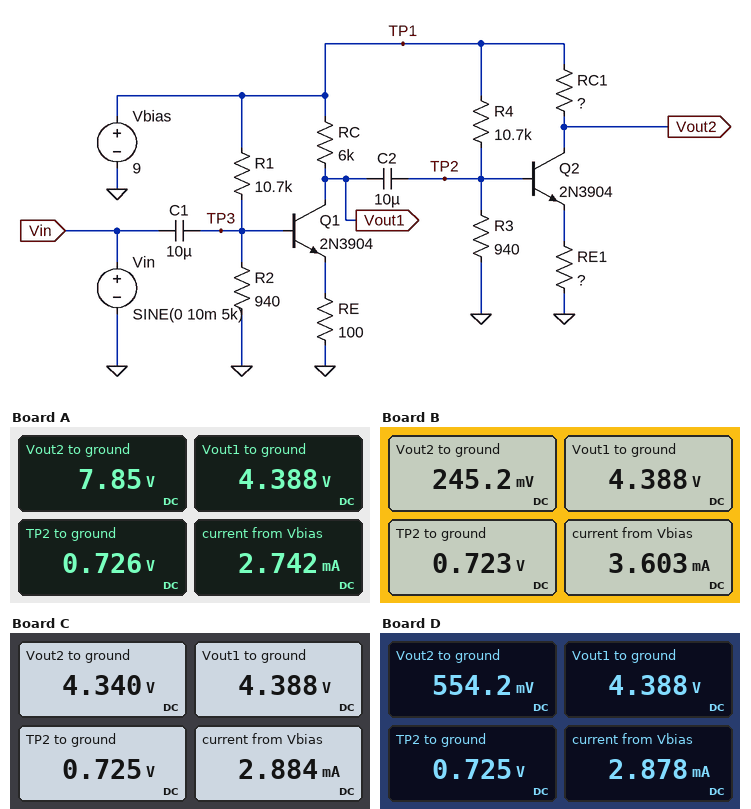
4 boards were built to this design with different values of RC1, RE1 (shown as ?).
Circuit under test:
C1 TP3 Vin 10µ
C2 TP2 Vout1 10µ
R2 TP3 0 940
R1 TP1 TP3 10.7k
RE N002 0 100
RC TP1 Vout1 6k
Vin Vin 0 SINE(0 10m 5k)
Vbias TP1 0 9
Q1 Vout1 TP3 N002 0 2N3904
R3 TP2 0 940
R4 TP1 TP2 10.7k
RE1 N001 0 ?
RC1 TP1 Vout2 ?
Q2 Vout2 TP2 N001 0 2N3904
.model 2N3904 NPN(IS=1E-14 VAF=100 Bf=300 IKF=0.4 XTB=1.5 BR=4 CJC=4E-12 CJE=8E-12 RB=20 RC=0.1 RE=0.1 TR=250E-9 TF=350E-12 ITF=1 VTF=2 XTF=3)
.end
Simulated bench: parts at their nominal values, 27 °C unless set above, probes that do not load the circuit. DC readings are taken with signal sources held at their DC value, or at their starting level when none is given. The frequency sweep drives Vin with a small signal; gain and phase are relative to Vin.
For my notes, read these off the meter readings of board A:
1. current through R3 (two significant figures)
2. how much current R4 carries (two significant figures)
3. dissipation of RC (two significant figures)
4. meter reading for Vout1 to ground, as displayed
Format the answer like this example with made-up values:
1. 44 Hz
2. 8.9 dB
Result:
1. 770 µA
2. 770 µA
3. 3.5 mW
4. 4.388 V
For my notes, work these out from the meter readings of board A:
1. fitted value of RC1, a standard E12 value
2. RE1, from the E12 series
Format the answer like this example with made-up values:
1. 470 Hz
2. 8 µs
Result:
1. 2.7 kΩ
2. 220 Ω
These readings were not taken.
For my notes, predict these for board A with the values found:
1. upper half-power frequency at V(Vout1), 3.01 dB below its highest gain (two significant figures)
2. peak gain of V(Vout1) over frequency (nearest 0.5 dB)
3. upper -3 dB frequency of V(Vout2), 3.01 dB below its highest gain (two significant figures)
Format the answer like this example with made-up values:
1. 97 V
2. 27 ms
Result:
1. 6.9 MHz
2. 15.0 dB
3. 6.5 MHz
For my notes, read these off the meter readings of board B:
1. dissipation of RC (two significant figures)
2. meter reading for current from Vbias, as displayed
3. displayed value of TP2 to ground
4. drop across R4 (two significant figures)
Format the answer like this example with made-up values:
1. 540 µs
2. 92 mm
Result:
1. 3.5 mW
2. 3.603 mA
3. 0.723 V
4. 8.3 V
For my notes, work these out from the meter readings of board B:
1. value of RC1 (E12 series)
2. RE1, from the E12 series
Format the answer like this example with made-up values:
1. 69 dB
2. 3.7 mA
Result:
1. 6.8 kΩ
2. 47 Ω
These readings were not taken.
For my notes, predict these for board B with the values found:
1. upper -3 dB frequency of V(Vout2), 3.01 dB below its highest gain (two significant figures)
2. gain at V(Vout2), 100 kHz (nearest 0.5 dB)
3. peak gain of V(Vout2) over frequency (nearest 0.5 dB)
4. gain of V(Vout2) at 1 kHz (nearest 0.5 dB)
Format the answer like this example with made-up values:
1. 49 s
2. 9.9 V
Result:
1. 240 kHz
2. 48.0 dB
3. 49.0 dB
4. 49.0 dB
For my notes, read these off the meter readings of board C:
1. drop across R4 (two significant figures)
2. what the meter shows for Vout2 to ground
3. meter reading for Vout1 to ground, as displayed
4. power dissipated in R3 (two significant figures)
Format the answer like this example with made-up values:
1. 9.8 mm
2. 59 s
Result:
1. 8.3 V
2. 4.340 V
3. 4.388 V
4. 560 µW
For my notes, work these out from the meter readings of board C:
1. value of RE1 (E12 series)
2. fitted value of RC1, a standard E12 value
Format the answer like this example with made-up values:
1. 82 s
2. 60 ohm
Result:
1. 150 Ω
2. 8.2 kΩ
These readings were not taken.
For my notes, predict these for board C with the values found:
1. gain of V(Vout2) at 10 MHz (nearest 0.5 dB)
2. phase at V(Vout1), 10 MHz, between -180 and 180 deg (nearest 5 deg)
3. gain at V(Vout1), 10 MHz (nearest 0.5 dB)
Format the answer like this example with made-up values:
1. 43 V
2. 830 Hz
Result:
1. 31.5 dB
2. 145 deg
3. 3.5 dB
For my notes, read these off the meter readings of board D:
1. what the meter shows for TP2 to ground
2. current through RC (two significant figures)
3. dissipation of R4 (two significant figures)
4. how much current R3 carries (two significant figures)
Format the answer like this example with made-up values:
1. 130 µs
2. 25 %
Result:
1. 0.725 V
2. 770 µA
3. 6.4 mW
4. 770 µA
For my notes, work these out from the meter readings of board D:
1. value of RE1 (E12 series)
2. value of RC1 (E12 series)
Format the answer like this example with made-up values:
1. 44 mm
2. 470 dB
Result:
1. 150 Ω
2. 15 kΩ
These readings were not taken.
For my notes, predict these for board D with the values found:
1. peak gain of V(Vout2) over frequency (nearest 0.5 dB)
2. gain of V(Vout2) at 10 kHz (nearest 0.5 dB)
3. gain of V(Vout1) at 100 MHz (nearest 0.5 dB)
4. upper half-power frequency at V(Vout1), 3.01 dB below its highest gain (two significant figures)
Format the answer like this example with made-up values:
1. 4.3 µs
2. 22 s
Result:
1. 52.5 dB
2. 52.5 dB
3. 1.0 dB
4. 520 kHz
